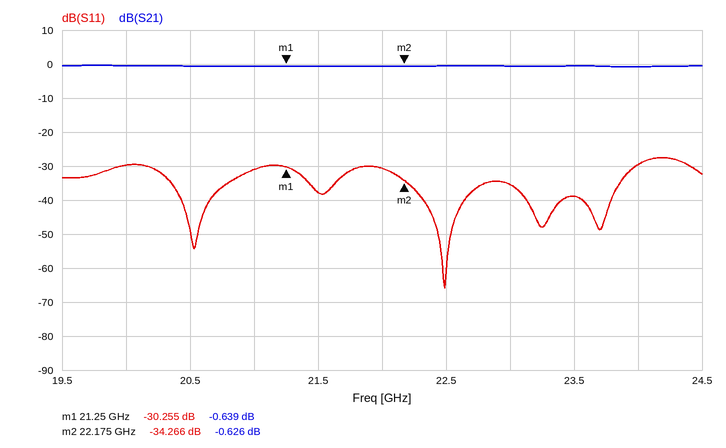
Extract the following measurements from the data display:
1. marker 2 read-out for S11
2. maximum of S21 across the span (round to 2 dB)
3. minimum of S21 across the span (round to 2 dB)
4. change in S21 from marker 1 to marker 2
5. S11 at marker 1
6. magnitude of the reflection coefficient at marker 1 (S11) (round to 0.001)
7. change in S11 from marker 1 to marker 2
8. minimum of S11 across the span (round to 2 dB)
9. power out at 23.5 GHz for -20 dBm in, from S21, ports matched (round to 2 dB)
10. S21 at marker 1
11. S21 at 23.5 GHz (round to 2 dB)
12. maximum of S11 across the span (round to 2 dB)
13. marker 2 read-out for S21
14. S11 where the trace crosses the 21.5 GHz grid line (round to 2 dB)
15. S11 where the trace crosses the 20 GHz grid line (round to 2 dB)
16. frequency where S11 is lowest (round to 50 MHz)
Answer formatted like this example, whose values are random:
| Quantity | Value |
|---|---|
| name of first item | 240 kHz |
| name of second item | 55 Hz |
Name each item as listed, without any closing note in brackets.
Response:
| Quantity | Value |
|---|---|
| marker 2 read-out for S11 | -34.266 dB |
| maximum of S21 across the span | 0 dB |
| minimum of S21 across the span | 0 dB |
| change in S21 from marker 1 to marker 2 | 0.013 dB |
| S11 at marker 1 | -30.255 dB |
| magnitude of the reflection coefficient at marker 1 (S11) | 0.031 |
| change in S11 from marker 1 to marker 2 | -4.011 dB |
| minimum of S11 across the span | -66 dB |
| power out at 23.5 GHz for -20 dBm in, from S21, ports matched | -20 dBm |
| S21 at marker 1 | -0.639 dB |
| S21 at 23.5 GHz | 0 dB |
| maximum of S11 across the span | -28 dB |
| marker 2 read-out for S21 | -0.626 dB |
| S11 where the trace crosses the 21.5 GHz grid line | -38 dB |
| S11 where the trace crosses the 20 GHz grid line | -30 dB |
| frequency where S11 is lowest | 22.50 GHz |
